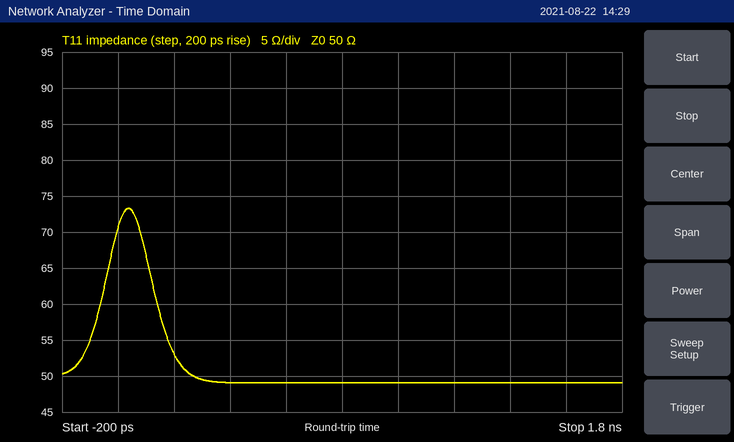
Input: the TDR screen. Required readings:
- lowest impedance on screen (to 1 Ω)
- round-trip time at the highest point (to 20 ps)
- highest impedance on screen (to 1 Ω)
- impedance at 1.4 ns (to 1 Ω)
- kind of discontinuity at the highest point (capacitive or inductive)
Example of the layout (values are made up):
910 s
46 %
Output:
49 Ω
40 ps
73 Ω
49 Ω
inductive
